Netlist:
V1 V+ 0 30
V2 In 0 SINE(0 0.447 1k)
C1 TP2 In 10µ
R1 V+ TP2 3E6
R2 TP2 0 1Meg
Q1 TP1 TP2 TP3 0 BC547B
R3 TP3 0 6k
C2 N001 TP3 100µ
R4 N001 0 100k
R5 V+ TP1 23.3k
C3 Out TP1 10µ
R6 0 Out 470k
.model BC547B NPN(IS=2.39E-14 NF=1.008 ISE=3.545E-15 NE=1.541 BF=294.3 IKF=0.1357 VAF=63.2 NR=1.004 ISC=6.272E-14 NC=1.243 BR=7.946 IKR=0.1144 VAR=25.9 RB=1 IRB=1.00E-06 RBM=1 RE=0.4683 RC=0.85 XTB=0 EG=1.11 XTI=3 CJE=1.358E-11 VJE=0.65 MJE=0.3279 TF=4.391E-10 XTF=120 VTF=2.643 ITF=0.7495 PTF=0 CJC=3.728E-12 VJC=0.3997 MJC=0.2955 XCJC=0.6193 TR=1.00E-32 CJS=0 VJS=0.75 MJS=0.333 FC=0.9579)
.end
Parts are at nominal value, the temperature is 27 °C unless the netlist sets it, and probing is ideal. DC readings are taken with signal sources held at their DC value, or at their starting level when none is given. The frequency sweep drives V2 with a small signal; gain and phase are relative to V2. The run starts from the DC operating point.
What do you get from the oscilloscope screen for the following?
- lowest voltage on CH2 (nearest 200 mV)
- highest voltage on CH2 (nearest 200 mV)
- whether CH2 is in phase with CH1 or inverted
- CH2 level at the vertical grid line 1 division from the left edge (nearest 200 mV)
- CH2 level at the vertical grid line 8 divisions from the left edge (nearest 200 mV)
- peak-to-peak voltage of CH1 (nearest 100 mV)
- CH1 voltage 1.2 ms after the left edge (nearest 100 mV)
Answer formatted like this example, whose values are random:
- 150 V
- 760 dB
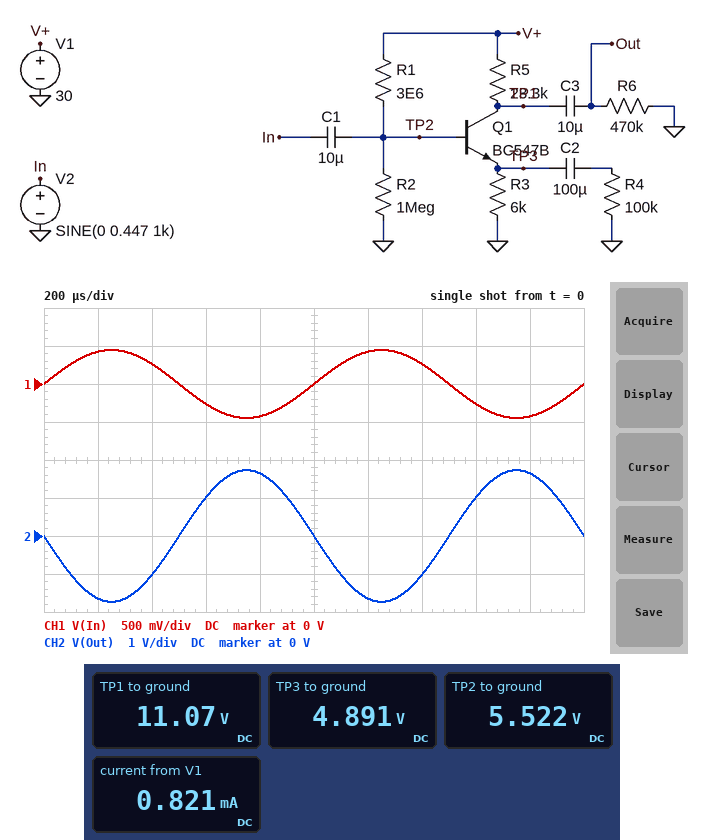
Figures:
- -1.8 V
- 1.8 V
- inverted
- -1.6 V
- 1.0 V
- 900 mV
- 400 mV
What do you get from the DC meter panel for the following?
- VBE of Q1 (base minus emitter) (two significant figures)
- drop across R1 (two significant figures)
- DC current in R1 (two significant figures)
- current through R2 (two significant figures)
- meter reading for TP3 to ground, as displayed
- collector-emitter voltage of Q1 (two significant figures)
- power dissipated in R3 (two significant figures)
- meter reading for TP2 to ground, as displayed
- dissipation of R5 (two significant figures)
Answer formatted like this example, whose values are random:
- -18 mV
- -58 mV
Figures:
- 630 mV
- 24 V
- 8.2 µA
- 5.5 µA
- 4.891 V
- 6.2 V
- 4.0 mW
- 5.522 V
- 15 mW
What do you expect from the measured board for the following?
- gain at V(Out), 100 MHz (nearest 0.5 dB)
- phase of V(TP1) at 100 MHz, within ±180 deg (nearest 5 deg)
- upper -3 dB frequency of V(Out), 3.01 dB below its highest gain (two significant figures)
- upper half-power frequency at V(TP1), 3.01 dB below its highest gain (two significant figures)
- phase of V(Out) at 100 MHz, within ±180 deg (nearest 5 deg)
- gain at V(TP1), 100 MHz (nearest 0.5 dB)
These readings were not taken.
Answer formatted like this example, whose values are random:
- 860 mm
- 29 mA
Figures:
- 0.5 dB
- 5 deg
- 4.7 MHz
- 4.7 MHz
- 5 deg
- 0.5 dB
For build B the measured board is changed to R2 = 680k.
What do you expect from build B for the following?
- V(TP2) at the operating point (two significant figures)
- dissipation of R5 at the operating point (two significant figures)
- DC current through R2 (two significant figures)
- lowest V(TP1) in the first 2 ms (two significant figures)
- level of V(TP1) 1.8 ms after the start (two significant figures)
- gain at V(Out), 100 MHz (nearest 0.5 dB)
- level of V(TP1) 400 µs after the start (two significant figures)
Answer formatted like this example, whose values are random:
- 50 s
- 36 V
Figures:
- 4.5 V
- 9.5 mW
- 6.6 µA
- 13 V
- 17 V
- 1.0 dB
- 14 V
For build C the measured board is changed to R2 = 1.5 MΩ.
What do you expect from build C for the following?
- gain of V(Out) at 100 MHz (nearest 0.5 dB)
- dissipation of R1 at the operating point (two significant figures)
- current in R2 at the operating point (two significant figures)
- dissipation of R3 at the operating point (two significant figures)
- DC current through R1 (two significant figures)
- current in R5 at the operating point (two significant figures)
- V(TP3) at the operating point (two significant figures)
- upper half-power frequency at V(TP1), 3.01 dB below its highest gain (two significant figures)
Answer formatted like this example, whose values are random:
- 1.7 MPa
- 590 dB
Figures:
- 0.5 dB
- 180 µW
- 4.4 µA
- 5.8 mW
- 7.8 µA
- 980 µA
- 5.9 V
- 2.7 MHz
